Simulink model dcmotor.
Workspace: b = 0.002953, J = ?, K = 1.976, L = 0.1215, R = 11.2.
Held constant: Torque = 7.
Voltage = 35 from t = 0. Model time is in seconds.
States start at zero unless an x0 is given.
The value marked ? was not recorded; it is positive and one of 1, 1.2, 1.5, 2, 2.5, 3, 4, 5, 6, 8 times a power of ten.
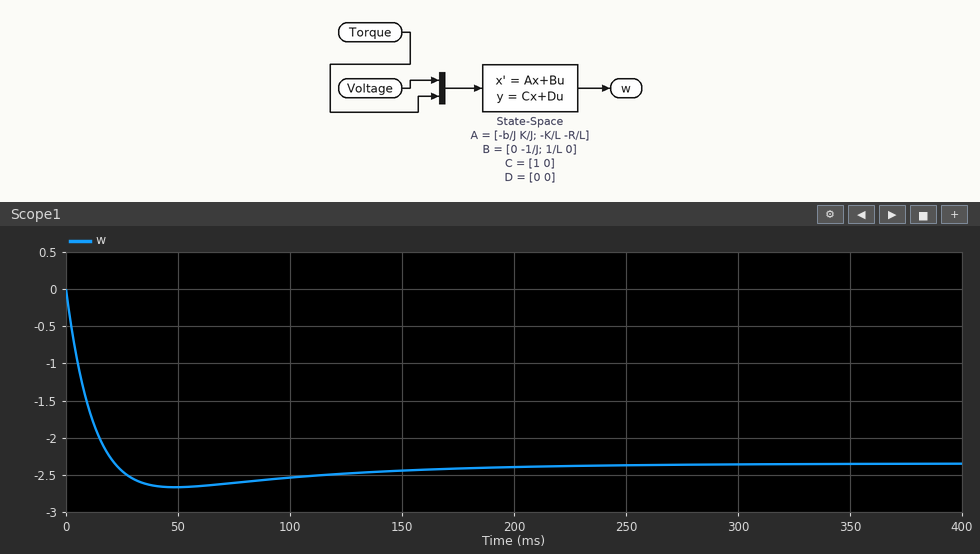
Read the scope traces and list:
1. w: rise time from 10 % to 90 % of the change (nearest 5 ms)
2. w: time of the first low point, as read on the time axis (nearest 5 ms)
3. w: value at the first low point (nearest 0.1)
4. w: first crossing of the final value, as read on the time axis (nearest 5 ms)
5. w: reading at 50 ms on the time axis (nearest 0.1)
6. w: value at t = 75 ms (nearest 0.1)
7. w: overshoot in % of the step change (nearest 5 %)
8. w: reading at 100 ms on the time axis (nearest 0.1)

15 ms
50 ms
-2.7
20 ms
-2.7
-2.6
15 %
-2.5
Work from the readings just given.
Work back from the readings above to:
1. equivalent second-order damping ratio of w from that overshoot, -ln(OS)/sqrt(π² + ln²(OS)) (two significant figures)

0.52
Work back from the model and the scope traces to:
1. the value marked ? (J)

0.03
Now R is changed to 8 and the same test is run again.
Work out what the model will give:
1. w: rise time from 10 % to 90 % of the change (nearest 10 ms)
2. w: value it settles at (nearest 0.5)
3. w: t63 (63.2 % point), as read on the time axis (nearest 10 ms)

90 ms
3.5
110 ms
